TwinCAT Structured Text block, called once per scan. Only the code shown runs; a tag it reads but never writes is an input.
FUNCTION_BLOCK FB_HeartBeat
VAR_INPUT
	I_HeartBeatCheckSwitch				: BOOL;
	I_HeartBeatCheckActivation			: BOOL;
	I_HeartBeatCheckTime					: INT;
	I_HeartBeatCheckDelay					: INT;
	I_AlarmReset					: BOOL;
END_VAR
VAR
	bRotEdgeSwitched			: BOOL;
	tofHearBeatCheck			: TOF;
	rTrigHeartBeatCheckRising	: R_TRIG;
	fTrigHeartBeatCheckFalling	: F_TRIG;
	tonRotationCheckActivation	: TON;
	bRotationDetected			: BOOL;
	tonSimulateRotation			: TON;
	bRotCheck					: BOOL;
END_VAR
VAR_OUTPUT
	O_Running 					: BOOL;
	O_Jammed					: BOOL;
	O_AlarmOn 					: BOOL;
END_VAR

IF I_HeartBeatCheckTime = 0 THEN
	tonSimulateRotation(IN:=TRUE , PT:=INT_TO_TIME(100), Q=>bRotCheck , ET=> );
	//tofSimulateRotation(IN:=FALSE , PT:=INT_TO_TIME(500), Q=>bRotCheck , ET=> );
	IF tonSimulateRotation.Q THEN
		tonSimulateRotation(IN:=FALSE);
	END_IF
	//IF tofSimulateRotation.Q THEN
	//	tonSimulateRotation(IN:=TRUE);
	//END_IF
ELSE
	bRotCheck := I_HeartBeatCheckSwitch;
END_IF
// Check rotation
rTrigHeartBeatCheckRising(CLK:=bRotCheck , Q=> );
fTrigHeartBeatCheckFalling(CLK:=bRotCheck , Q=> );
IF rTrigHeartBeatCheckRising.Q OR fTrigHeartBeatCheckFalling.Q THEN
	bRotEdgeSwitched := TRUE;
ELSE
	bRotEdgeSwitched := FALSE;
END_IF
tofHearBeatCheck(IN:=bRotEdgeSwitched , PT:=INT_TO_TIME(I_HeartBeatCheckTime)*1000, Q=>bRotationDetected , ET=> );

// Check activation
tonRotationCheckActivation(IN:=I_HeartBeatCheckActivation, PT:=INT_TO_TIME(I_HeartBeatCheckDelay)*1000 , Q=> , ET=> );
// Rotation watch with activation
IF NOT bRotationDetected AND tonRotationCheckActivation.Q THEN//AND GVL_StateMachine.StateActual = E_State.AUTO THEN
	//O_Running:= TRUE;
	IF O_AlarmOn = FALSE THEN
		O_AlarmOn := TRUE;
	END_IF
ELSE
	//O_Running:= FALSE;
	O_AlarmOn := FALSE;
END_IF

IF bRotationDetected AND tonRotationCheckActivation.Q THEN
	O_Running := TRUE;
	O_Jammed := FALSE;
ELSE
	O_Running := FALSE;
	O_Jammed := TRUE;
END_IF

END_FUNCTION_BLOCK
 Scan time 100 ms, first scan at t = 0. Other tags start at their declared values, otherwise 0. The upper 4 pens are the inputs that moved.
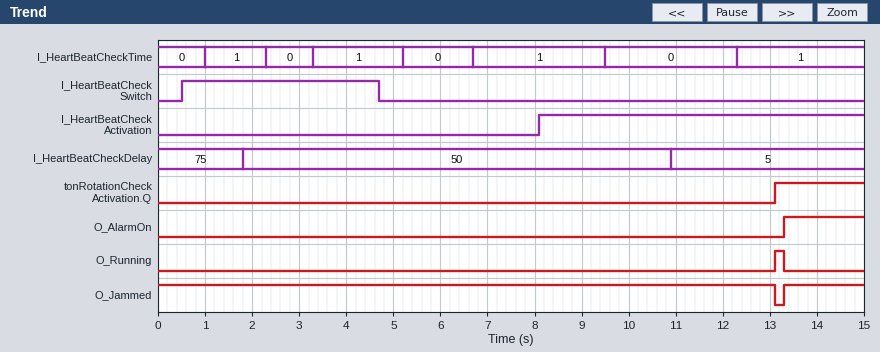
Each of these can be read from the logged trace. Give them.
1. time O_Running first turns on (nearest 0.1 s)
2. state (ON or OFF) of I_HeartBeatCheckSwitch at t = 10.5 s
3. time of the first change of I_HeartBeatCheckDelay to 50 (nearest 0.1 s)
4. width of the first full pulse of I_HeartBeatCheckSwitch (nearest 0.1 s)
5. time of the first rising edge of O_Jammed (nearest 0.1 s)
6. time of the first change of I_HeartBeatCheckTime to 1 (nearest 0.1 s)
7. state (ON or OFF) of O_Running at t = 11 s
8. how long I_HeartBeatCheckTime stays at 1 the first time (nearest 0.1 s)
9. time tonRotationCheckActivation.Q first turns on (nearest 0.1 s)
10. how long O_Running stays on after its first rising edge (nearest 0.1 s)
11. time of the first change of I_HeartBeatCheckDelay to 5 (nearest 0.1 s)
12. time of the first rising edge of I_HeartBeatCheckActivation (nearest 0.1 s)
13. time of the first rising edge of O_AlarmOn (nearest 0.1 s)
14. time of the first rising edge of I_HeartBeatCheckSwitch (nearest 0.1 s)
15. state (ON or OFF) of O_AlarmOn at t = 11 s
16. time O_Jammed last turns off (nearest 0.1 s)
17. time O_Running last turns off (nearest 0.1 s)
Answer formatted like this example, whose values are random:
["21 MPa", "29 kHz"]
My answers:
["13.1 s", "OFF", "1.8 s", "4.2 s", "13.3 s", "1.0 s", "OFF", "1.3 s", "13.1 s", "0.2 s", "10.9 s", "8.1 s", "13.3 s", "0.5 s", "OFF", "13.1 s", "13.3 s"]
